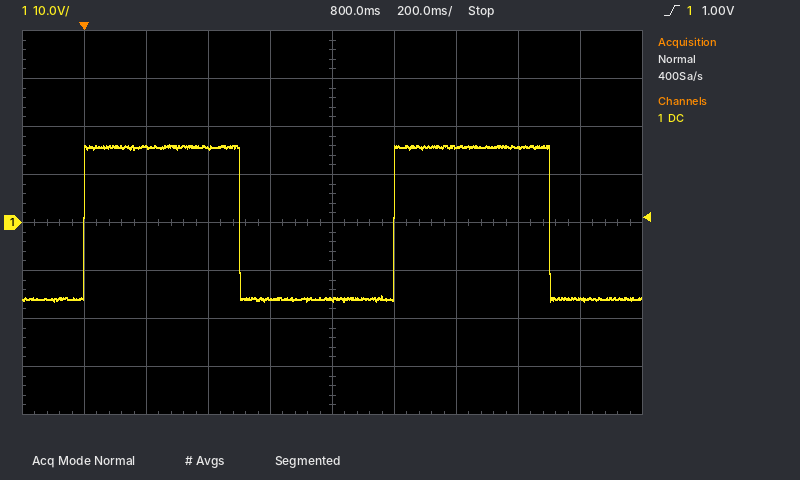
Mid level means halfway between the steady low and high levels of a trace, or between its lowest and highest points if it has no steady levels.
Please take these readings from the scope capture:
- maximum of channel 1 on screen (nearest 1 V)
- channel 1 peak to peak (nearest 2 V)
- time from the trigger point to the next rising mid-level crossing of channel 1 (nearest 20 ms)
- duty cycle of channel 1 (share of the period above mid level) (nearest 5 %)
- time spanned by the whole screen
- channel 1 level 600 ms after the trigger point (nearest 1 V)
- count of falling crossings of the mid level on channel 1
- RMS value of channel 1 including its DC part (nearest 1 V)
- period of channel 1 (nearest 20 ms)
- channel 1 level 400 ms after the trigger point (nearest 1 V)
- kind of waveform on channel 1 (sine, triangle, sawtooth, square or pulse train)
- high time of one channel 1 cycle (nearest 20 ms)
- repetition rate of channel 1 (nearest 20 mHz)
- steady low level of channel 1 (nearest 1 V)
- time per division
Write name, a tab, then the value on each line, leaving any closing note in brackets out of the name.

maximum of channel 1 on screen	16 V
channel 1 peak to peak	32 V
time from the trigger point to the next rising mid-level crossing of channel 1	1.00 s
duty cycle of channel 1 (share of the period above mid level)	50 %
time spanned by the whole screen	2 s
channel 1 level 600 ms after the trigger point	-16 V
count of falling crossings of the mid level on channel 1	2
RMS value of channel 1 including its DC part	16 V
period of channel 1	1.00 s
channel 1 level 400 ms after the trigger point	16 V
kind of waveform on channel 1	square
high time of one channel 1 cycle	500 ms
repetition rate of channel 1	1.00 Hz
steady low level of channel 1	-16 V
time per division	200 ms
